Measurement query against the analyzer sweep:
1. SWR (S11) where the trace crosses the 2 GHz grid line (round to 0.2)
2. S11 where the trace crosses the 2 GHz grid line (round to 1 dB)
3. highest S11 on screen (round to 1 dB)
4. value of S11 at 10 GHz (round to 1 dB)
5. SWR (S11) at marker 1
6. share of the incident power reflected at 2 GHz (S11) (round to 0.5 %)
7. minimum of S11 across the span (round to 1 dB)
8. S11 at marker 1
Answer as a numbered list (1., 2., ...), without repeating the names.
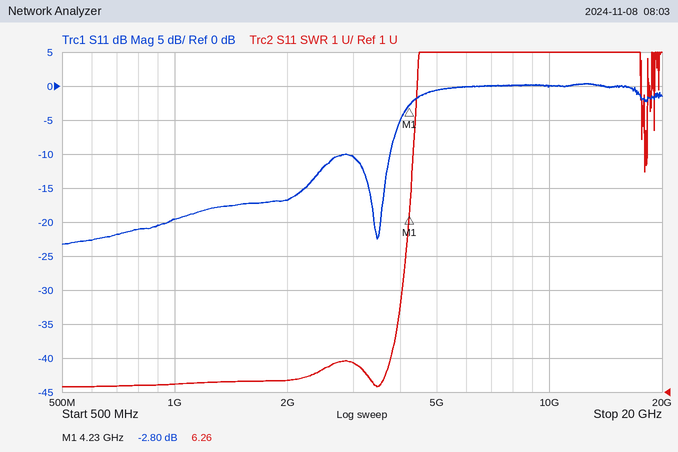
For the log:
1. 1.4
2. -17 dB
3. 0 dB
4. 0 dB
5. 6.26
6. 2.0 %
7. -23 dB
8. -2.80 dB
